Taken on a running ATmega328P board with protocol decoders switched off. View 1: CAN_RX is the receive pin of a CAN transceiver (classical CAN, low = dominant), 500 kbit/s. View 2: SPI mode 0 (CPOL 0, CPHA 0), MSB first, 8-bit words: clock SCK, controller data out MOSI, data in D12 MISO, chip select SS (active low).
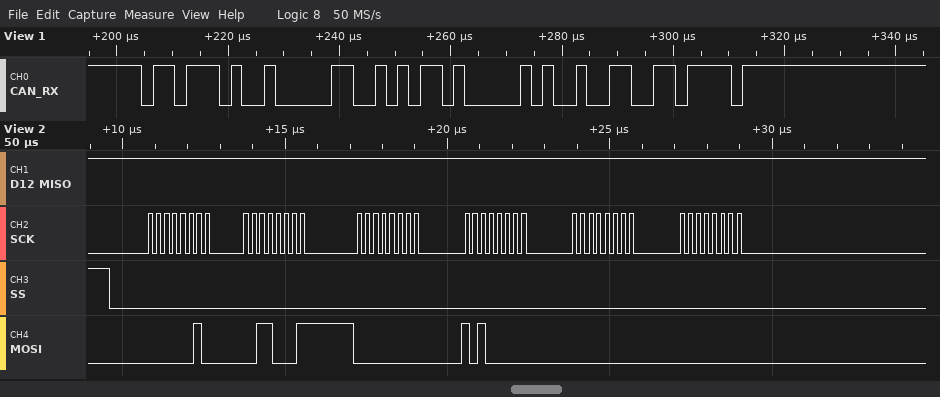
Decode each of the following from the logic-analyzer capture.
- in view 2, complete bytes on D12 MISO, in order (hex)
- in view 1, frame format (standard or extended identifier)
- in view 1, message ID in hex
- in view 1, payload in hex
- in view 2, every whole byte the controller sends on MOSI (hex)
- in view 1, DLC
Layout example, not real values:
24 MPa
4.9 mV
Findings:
FF FF FF FF FF FF
standard
0x6E9
56 81
02 31 00 A0 00 00
2
